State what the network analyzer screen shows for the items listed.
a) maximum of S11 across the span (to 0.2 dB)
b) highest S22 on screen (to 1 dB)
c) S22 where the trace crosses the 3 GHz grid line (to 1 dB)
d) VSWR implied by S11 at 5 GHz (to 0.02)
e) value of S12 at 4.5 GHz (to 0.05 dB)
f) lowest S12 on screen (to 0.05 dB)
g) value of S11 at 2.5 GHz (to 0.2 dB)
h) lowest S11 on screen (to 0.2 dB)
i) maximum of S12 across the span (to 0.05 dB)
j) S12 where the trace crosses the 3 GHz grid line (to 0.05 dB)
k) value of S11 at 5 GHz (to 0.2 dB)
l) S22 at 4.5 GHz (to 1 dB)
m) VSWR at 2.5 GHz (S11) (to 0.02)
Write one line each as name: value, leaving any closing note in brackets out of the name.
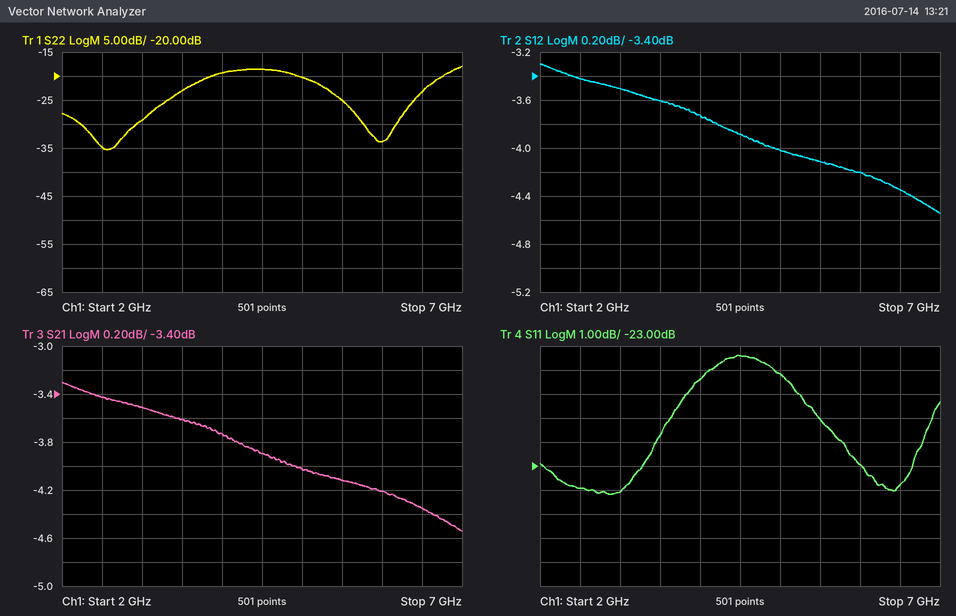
maximum of S11 across the span: -18.4 dB
highest S22 on screen: -18 dB
S22 where the trace crosses the 3 GHz grid line: -29 dB
VSWR implied by S11 at 5 GHz: 1.24
value of S12 at 4.5 GHz: -3.90 dB
lowest S12 on screen: -4.55 dB
value of S11 at 2.5 GHz: -24.0 dB
lowest S11 on screen: -24.2 dB
maximum of S12 across the span: -3.30 dB
S12 where the trace crosses the 3 GHz grid line: -3.50 dB
value of S11 at 5 GHz: -19.2 dB
S22 at 4.5 GHz: -19 dB
VSWR at 2.5 GHz (S11): 1.14
